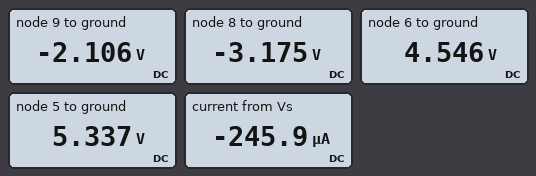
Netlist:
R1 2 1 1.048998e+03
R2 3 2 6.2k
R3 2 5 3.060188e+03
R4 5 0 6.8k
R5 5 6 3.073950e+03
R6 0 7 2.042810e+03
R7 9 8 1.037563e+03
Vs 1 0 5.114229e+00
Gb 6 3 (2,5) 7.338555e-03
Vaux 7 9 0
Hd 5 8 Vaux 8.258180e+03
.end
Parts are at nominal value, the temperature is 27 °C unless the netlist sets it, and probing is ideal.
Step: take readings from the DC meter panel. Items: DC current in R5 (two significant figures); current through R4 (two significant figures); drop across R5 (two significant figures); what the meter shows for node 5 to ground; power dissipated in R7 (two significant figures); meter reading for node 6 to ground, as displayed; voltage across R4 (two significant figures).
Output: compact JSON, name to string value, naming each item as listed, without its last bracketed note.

{"DC current in R5": "260 µA", "current through R4": "780 µA", "drop across R5": "790 mV", "what the meter shows for node 5 to ground": "5.337 V", "power dissipated in R7": "1.1 mW", "meter reading for node 6 to ground, as displayed": "4.546 V", "voltage across R4": "5.3 V"}
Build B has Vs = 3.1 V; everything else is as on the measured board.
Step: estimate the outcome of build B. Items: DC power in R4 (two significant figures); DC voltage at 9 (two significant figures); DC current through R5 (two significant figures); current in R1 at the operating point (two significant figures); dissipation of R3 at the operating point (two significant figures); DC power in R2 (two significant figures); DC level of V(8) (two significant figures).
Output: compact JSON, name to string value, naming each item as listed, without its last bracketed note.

{"DC power in R4": "1.5 mW", "DC voltage at 9": "-1.3 V", "DC current through R5": "160 µA", "current in R1 at the operating point": "150 µA", "dissipation of R3 at the operating point": "150 nW", "DC power in R2": "150 µW", "DC level of V(8)": "-1.9 V"}
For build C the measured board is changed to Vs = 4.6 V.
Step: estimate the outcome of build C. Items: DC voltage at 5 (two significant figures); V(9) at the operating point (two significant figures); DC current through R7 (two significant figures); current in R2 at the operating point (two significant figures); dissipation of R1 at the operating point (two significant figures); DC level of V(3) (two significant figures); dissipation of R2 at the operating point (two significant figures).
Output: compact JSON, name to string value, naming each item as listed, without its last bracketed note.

{"DC voltage at 5": "4.8 V", "V(9) at the operating point": "-1.9 V", "DC current through R7": "930 µA", "current in R2 at the operating point": "230 µA", "dissipation of R1 at the operating point": "51 µW", "DC level of V(3)": "6.3 V", "dissipation of R2 at the operating point": "330 µW"}
